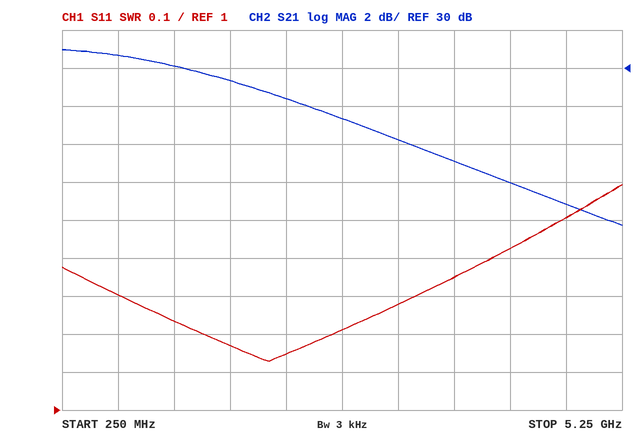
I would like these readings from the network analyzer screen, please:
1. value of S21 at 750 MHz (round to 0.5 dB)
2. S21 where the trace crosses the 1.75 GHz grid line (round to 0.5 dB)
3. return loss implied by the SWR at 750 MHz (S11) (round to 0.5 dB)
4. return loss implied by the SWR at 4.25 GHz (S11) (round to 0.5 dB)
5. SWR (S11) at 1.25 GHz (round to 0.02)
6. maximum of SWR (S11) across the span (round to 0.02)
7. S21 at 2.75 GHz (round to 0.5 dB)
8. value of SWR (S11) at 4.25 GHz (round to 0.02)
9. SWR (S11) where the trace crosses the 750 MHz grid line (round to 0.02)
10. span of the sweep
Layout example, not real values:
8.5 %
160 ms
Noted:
30.5 dB
29.5 dB
17.5 dB
15.0 dB
1.24
1.60
27.5 dB
1.42
1.30
5 GHz
